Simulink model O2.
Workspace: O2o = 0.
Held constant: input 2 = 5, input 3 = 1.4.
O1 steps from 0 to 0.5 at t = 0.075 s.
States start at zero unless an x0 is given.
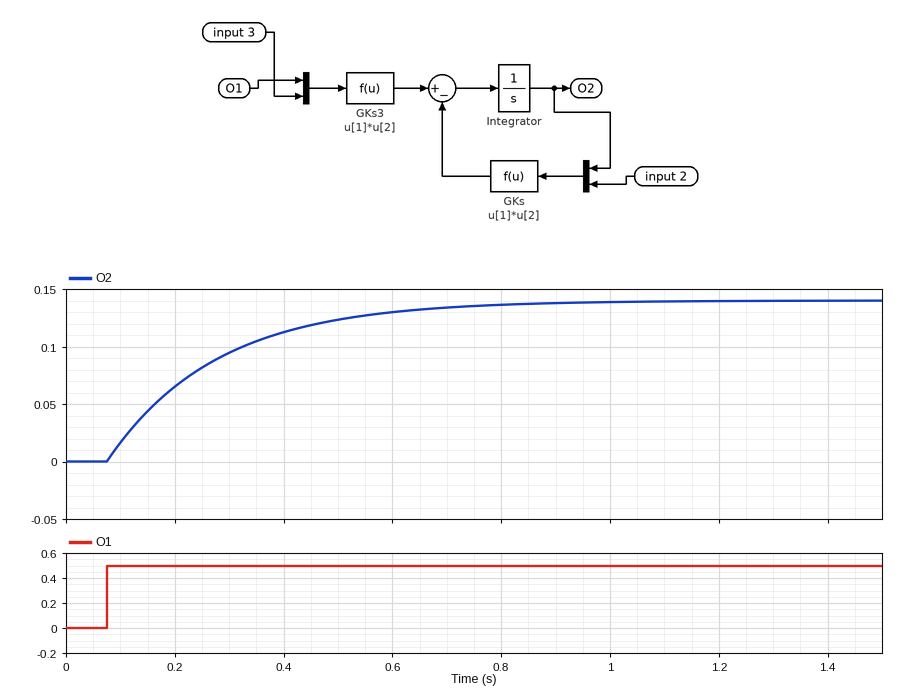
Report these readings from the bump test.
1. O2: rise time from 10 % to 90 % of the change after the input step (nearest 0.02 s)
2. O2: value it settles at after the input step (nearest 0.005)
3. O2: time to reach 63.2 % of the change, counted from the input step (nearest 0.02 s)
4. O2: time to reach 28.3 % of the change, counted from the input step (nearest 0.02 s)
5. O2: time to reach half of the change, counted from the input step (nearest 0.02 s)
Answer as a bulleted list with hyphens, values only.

- 0.44 s
- 0.140
- 0.20 s
- 0.06 s
- 0.14 s
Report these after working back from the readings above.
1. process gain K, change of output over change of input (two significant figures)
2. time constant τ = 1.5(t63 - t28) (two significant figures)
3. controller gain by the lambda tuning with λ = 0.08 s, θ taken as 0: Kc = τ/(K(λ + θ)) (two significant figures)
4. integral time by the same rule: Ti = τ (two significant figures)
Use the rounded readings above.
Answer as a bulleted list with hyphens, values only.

- 0.28
- 0.21 s
- 9.4
- 0.21 s
